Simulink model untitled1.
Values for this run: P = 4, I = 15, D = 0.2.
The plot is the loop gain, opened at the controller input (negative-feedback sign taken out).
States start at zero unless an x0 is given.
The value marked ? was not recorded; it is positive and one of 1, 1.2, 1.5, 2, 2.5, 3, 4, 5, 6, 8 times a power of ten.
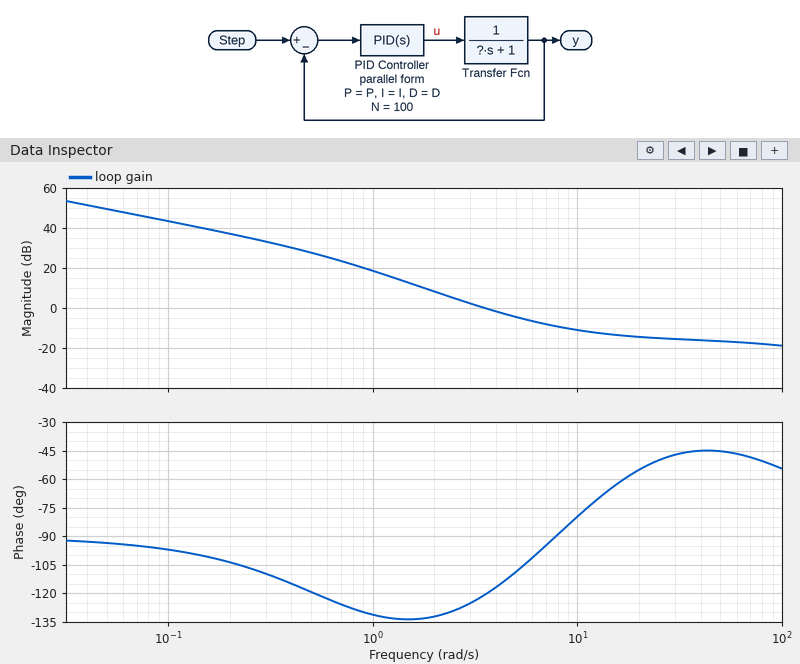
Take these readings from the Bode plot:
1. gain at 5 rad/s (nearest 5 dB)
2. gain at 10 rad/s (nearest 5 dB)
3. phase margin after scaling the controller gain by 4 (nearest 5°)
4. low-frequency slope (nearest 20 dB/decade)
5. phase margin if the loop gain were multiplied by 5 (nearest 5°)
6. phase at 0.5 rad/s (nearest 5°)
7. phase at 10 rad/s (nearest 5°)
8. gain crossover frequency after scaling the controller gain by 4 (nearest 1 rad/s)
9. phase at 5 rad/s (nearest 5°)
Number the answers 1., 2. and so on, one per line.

1. -5 dB
2. -10 dB
3. 105°
4. -20 dB/decade
5. 120°
6. -120°
7. -80°
8. 12 rad/s
9. -110°
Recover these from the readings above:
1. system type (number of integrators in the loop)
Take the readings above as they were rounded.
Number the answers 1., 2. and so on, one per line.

1. 1
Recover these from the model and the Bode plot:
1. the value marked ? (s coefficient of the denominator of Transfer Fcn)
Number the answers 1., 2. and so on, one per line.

1. 1.5
